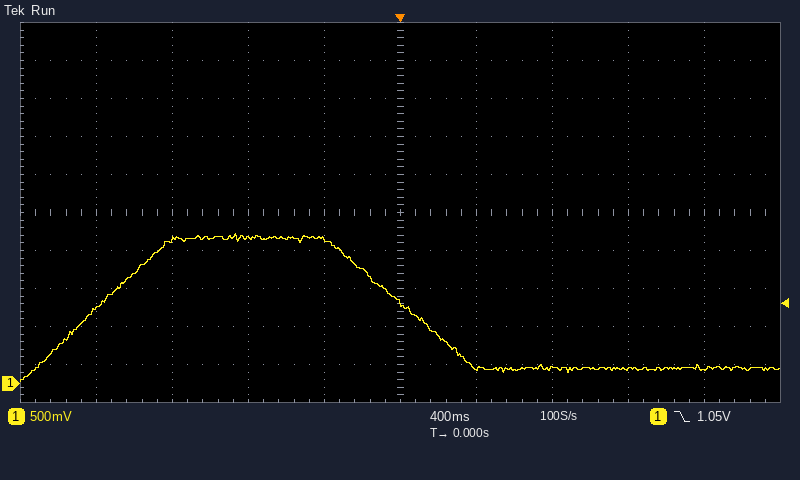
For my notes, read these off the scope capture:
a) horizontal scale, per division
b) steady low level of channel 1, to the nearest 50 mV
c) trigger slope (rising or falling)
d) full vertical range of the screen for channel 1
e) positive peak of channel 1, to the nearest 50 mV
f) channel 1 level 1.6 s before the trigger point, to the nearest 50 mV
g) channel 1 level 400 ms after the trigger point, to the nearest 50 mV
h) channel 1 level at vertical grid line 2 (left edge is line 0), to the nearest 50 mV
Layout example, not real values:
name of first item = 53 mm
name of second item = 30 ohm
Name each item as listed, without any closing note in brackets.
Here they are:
horizontal scale, per division = 400 ms
steady low level of channel 1, to the nearest 50 mV = 200 mV
trigger slope = falling
full vertical range of the screen for channel 1 = 5 V
positive peak of channel 1, to the nearest 50 mV = 1.95 V
channel 1 level 1.6 s before the trigger point, to the nearest 50 mV = 1.00 V
channel 1 level 400 ms after the trigger point, to the nearest 50 mV = 200 mV
channel 1 level at vertical grid line 2 (left edge is line 0), to the nearest 50 mV = 1.90 V
